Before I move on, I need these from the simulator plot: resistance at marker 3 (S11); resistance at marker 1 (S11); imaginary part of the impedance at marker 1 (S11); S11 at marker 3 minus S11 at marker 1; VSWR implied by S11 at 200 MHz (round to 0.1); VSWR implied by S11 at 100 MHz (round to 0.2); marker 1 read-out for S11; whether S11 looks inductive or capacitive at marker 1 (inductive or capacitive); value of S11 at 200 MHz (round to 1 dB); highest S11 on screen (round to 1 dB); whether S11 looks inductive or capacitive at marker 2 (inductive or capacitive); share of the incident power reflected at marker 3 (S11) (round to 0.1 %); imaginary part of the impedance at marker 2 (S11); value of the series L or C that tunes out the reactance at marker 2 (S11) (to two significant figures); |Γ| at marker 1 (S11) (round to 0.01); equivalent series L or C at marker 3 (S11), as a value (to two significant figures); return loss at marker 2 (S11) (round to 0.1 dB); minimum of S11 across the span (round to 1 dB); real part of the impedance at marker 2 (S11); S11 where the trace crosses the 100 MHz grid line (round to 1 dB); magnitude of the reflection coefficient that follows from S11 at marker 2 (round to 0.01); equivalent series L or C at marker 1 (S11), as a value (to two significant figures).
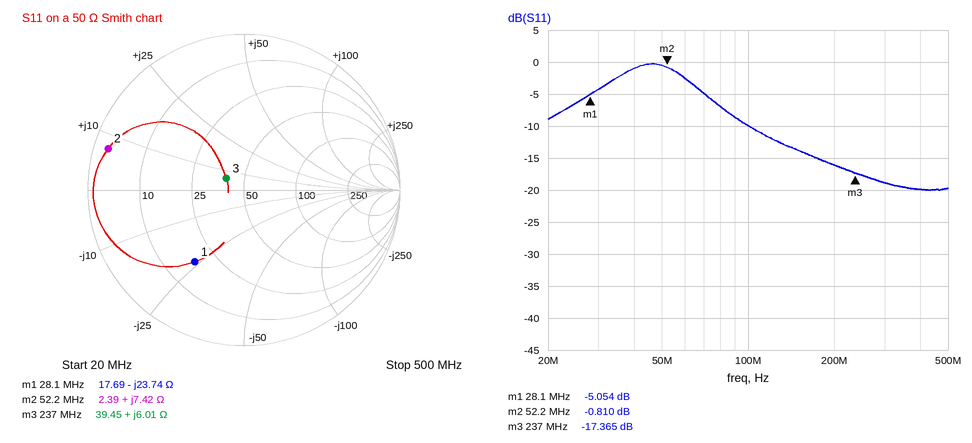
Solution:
39.45 Ω
17.69 Ω
-23.74 Ω
-12.311 dB
1.4
2.0
-5.054 dB
capacitive
-16 dB
0 dB
inductive
1.8 %
+7.42 Ω
410 pF
0.56
4.0 nH
0.8 dB
-20 dB
2.39 Ω
-10 dB
0.91
240 pF
